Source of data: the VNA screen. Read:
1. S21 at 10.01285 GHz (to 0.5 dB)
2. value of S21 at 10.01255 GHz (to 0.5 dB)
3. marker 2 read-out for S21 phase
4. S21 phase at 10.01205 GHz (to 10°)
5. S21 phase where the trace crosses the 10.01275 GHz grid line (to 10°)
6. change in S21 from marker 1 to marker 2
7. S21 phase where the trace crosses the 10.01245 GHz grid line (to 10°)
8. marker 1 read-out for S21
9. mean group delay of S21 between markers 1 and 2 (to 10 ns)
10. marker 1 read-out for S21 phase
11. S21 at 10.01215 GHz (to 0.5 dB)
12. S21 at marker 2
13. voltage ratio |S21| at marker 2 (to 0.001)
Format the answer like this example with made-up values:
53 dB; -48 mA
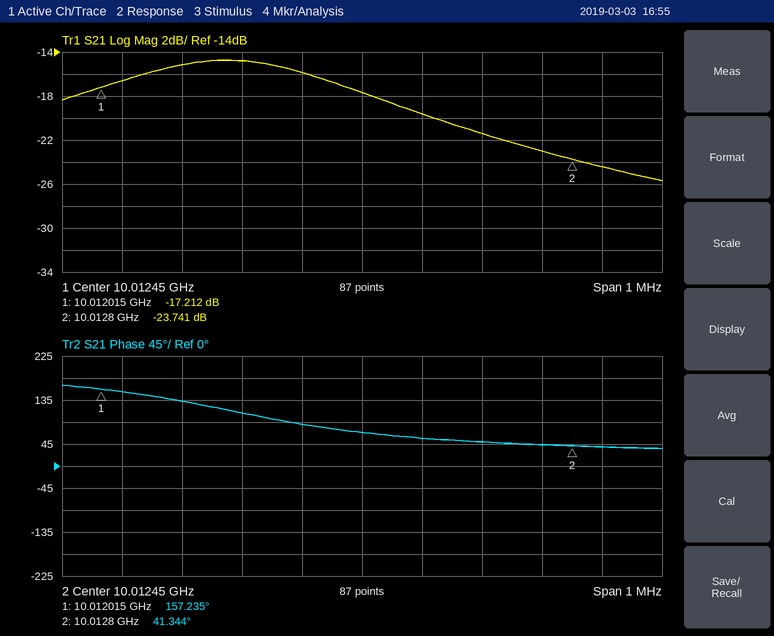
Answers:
-24.5 dB; -19.5 dB; 41.344°; 150°; 40°; -6.529 dB; 70°; -17.212 dB; 410 ns; 157.235°; -15.0 dB; -23.741 dB; 0.065
